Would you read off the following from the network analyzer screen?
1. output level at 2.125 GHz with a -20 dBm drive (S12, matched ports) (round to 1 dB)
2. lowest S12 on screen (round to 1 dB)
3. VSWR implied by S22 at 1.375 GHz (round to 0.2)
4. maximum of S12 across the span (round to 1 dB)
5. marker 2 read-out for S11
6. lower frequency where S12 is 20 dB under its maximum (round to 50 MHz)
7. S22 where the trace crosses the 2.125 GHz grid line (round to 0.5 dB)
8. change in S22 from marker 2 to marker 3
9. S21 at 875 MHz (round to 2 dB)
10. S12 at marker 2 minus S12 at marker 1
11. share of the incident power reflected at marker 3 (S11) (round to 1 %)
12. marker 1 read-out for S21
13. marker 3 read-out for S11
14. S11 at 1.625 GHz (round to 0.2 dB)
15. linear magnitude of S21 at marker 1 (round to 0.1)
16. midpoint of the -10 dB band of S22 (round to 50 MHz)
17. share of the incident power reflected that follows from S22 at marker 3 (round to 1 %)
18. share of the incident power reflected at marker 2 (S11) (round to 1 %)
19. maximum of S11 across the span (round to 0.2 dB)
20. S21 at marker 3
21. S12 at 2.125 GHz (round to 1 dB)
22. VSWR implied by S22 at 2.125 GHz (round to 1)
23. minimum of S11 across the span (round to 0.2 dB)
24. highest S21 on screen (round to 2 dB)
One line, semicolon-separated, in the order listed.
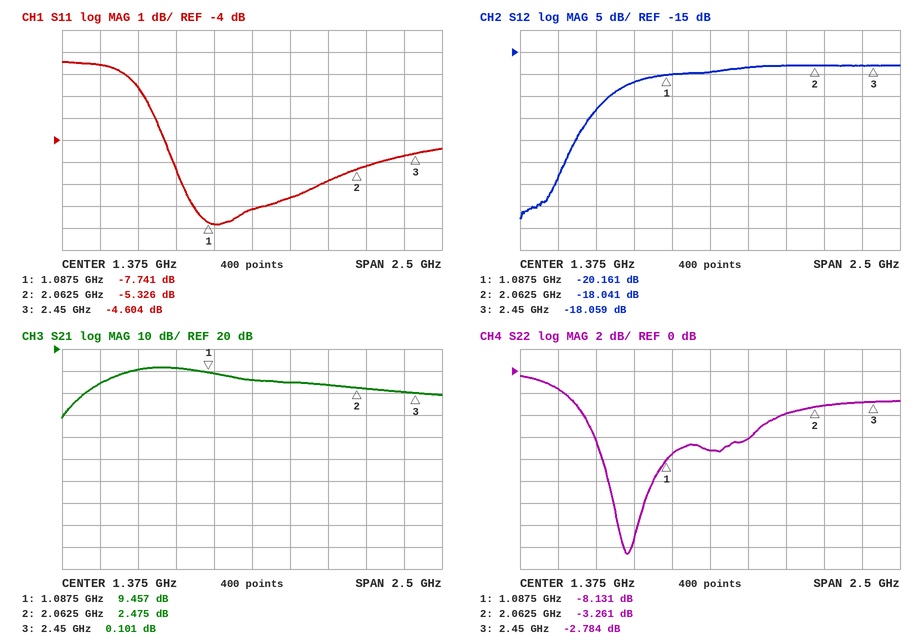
-38 dBm; -53 dB; 2.6; -18 dB; -5.326 dB; 450 MHz; -3.0 dB; 0.477 dB; 12 dB; 2.120 dB; 35 %; 9.457 dB; -4.604 dB; -6.6 dB; 3.0; 850 MHz; 53 %; 29 %; -0.4 dB; 0.101 dB; -18 dB; 6; -7.8 dB; 12 dB
